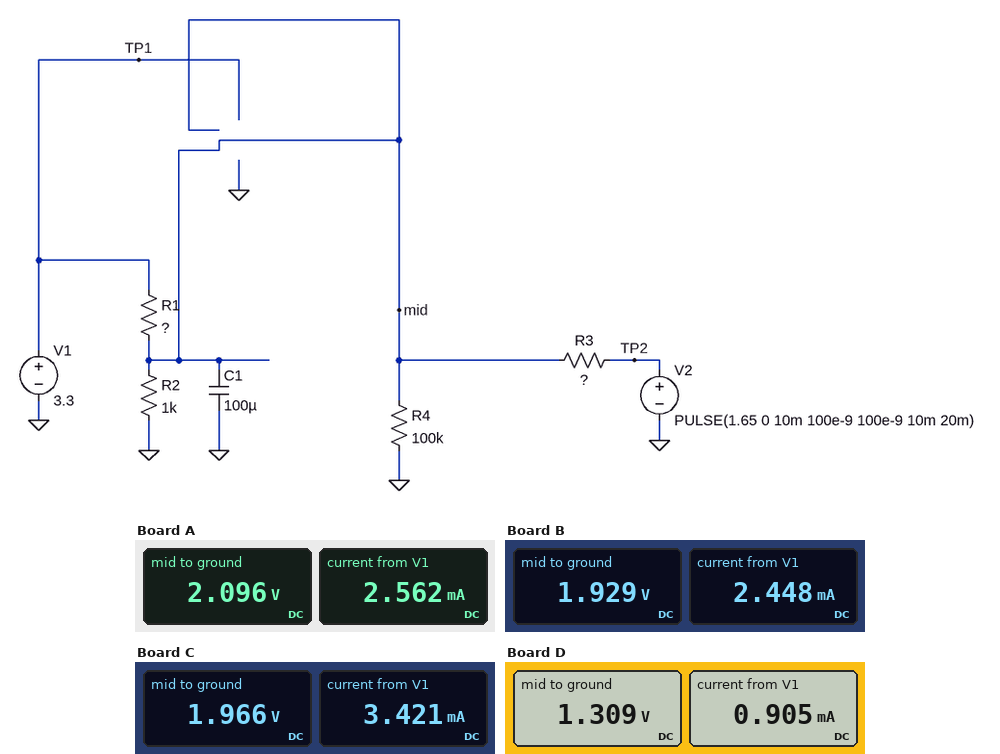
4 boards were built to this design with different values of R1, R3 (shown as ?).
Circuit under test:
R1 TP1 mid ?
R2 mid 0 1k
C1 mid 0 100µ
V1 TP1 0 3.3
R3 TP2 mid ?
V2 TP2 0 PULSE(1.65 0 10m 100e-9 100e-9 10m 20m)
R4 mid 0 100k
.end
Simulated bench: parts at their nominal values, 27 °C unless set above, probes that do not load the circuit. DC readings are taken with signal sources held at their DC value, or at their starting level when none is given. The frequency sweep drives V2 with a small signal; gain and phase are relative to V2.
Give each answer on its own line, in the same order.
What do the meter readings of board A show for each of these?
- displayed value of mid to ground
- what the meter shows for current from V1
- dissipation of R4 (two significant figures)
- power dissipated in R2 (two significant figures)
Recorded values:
2.096 V
2.562 mA
44 µW
4.4 mW
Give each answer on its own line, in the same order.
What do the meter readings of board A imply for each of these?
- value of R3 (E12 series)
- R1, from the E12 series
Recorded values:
1 kΩ
470 Ω
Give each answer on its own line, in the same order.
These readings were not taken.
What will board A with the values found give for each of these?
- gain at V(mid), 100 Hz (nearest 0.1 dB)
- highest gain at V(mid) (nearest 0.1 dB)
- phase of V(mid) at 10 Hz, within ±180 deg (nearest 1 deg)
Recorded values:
-36.0 dB
-12.3 dB
-57 deg
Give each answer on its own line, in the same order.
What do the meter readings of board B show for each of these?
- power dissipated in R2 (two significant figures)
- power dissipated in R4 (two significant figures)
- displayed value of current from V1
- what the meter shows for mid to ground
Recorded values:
3.7 mW
37 µW
2.448 mA
1.929 V
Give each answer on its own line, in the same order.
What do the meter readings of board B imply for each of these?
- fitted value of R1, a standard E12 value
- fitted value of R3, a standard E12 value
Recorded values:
560 Ω
560 Ω
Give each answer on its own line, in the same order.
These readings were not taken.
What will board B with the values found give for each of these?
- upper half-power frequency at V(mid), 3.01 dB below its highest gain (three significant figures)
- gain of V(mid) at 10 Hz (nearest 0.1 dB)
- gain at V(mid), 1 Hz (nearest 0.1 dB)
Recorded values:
7.29 Hz
-12.8 dB
-8.3 dB
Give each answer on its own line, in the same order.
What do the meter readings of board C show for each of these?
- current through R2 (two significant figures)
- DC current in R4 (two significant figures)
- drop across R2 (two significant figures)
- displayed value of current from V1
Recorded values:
2.0 mA
20 µA
2.0 V
3.421 mA
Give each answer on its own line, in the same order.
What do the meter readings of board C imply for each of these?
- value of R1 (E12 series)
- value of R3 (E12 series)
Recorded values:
390 Ω
220 Ω
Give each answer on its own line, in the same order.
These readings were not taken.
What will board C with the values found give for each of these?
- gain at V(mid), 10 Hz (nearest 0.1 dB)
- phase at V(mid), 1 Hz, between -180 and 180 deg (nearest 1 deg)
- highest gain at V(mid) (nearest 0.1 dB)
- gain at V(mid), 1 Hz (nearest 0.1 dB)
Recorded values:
-7.1 dB
-4 deg
-5.0 dB
-5.1 dB
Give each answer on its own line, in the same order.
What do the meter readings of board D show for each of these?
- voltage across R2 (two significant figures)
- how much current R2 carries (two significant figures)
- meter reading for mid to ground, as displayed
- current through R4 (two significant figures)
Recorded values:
1.3 V
1.3 mA
1.309 V
13 µA
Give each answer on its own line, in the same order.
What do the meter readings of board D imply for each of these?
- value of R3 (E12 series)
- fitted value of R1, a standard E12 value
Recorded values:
820 Ω
2.2 kΩ
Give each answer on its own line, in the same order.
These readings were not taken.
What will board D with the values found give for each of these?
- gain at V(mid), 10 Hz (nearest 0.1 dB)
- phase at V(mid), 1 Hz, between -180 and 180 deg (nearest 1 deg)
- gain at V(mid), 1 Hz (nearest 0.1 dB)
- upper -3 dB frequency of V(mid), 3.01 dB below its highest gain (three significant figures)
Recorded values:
-15.0 dB
-13 deg
-7.1 dB
4.27 Hz
